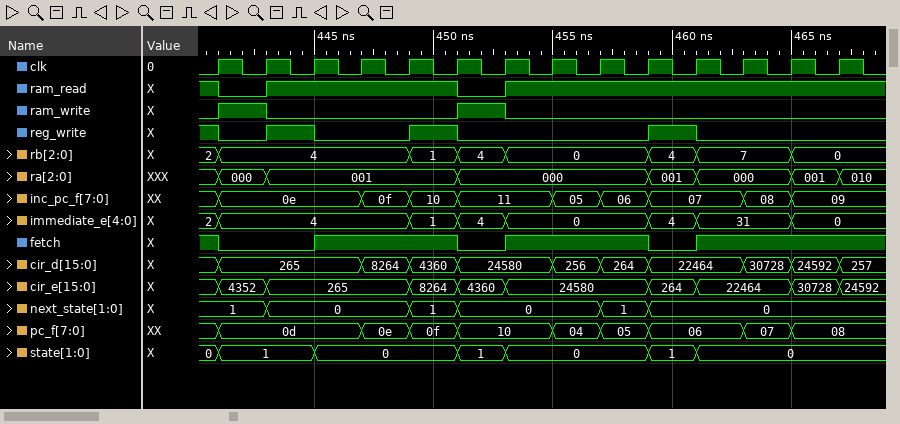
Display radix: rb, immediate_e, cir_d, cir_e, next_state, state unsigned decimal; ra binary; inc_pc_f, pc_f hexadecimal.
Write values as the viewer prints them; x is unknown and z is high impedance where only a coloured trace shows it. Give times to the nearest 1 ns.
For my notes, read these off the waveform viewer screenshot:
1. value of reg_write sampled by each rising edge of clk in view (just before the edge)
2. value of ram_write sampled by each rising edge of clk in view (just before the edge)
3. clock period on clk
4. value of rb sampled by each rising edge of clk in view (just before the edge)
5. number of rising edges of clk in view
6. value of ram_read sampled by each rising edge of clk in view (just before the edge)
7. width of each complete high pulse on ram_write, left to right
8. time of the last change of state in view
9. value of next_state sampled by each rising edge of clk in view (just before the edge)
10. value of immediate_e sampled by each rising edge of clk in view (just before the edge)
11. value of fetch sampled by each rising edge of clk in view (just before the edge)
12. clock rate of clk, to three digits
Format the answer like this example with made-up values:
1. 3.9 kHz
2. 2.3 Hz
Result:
1. 1 0 1 0 0 1 0 0 0 0 1 0 0 0
2. 0 1 0 0 0 0 1 0 0 0 0 0 0 0
3. 2 ns
4. 2, 4, 4, 4, 4, 1, 4, 0, 0, 0, 4, 7, 7, 0
5. 14
6. 1 0 1 1 1 1 0 1 1 1 1 1 1 1
7. 2 ns, 2 ns
8. 461 ns
9. 1, 1, 0, 0, 0, 1, 0, 0, 0, 1, 0, 0, 0, 0
10. 2, 4, 4, 4, 4, 1, 4, 0, 0, 0, 4, 31, 31, 0
11. 1 0 0 1 1 1 0 1 1 1 0 1 1 1
12. 500 MHz
